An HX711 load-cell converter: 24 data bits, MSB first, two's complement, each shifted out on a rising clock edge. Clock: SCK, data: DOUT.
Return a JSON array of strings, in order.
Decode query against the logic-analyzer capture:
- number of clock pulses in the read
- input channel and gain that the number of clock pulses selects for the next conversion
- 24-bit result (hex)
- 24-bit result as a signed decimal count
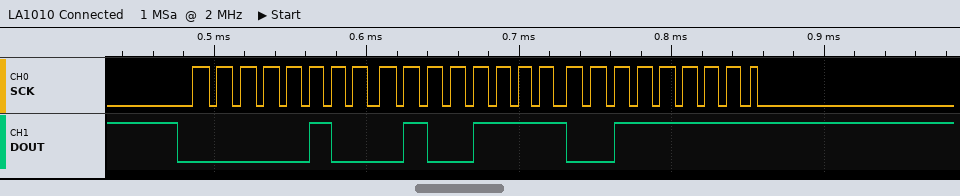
["25", "channel A, gain 128", "0x044F3F", "282431"]
